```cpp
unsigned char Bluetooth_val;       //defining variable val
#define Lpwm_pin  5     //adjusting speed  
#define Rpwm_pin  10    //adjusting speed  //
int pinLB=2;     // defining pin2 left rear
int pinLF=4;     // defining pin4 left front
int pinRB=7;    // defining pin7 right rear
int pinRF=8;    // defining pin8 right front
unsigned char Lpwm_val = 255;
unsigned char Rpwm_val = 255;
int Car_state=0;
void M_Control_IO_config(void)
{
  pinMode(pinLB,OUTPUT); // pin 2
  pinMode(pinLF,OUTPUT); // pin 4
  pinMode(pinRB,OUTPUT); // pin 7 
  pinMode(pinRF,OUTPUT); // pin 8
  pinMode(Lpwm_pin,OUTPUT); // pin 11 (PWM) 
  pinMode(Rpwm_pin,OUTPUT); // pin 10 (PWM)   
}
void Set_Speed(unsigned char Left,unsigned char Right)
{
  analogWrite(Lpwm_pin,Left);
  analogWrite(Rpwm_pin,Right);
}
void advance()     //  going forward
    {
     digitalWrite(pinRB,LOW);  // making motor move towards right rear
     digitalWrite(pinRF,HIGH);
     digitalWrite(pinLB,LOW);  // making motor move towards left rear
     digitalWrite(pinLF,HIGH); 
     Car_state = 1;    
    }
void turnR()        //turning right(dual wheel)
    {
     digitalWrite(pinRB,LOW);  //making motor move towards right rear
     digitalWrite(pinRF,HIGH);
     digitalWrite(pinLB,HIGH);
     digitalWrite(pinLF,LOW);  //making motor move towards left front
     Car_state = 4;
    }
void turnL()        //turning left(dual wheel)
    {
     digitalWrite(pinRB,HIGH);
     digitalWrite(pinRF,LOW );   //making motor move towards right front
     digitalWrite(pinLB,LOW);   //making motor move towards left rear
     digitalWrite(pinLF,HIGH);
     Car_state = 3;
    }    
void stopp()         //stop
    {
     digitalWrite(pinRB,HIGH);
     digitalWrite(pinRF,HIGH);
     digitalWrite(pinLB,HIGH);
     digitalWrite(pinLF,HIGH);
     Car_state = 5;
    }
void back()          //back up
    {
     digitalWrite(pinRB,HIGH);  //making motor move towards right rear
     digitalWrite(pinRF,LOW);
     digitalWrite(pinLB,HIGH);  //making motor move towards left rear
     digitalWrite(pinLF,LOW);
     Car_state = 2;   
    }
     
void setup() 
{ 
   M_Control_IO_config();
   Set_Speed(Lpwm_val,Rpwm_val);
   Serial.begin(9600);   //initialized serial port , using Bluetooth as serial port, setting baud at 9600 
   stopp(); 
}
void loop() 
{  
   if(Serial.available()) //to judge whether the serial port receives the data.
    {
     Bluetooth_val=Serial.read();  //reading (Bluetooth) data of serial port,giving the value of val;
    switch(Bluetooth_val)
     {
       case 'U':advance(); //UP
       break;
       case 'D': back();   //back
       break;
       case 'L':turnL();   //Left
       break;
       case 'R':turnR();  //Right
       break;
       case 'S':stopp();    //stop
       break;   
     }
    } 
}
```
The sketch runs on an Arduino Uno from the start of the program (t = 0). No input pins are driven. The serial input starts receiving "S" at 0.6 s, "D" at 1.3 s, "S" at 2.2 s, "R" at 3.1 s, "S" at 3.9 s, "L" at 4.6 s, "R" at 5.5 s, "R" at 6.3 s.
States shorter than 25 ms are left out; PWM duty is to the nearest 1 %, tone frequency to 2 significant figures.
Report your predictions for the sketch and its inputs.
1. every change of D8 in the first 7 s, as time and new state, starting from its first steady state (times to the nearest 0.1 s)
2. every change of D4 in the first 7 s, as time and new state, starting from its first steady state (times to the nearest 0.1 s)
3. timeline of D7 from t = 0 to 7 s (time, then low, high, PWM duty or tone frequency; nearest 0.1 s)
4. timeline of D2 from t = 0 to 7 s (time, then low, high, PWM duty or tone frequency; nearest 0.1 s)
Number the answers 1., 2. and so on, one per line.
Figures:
1. 0 s high; 1.3 s low; 2.2 s high; 4.6 s low; 5.5 s high
2. 0 s high; 1.3 s low; 2.2 s high; 3.1 s low; 3.9 s high; 5.5 s low
3. 0 s high; 3.1 s low; 3.9 s high; 5.5 s low
4. 0 s high; 4.6 s low; 5.5 s high
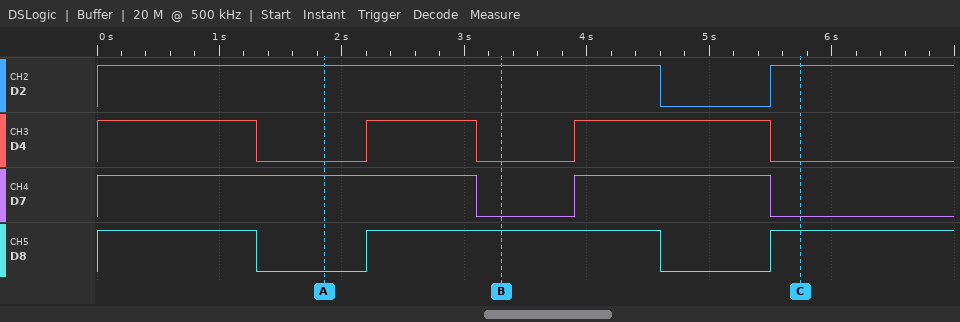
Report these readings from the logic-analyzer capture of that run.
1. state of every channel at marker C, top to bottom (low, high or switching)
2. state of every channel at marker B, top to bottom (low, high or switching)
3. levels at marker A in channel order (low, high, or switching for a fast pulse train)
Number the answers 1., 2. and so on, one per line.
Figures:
1. D2 high, D4 low, D7 low, D8 high
2. D2 high, D4 low, D7 low, D8 high
3. D2 high, D4 low, D7 high, D8 low
